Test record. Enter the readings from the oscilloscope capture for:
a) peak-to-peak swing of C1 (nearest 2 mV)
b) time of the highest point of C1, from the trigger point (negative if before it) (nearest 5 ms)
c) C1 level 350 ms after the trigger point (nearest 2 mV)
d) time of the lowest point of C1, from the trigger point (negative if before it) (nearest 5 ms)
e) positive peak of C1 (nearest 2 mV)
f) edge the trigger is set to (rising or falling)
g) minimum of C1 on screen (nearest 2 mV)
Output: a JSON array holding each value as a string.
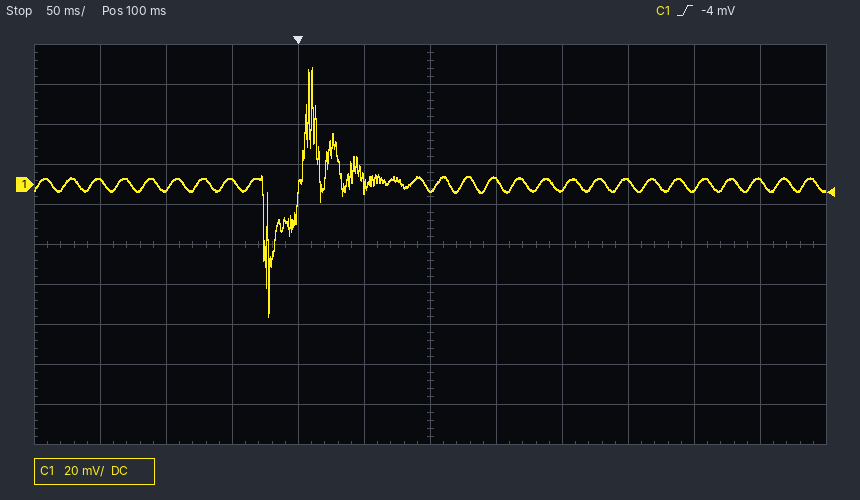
["124 mV", "+10 ms", "2 mV", "-20 ms", "58 mV", "rising", "-66 mV"]
